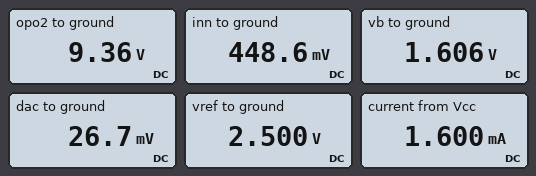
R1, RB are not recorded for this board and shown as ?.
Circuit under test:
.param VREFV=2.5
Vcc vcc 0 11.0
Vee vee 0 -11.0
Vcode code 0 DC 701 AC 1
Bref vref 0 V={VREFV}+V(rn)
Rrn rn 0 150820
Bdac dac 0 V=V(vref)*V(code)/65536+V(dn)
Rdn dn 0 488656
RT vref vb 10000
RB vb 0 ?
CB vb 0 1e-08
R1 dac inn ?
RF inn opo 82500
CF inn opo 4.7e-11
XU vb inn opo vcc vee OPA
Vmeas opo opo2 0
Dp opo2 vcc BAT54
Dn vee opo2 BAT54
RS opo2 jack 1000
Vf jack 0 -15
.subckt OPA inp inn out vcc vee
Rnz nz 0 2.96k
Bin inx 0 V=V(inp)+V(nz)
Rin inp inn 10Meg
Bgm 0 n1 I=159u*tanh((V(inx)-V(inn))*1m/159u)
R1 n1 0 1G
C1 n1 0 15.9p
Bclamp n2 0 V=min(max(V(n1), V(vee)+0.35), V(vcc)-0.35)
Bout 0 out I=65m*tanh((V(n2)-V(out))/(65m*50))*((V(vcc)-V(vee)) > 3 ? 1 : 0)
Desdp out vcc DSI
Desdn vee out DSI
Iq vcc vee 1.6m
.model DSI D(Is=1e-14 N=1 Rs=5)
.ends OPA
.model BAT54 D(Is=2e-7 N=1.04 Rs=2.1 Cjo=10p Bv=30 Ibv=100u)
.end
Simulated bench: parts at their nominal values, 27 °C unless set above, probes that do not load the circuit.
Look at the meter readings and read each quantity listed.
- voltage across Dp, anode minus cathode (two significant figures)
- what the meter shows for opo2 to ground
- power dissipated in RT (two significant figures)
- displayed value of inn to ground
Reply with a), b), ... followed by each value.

a) -1.6 V
b) 9.36 V
c) 80 µW
d) 448.6 mV
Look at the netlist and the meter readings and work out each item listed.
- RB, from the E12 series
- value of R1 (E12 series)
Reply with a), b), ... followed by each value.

a) 18 kΩ
b) 3.9 kΩ
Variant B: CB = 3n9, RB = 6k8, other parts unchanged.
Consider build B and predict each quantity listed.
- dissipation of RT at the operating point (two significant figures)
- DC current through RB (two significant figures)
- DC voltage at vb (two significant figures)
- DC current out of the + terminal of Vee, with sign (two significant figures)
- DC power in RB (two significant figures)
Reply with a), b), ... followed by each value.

a) 220 µW
b) 150 µA
c) 1.0 V
d) -1.6 mA
e) 150 µW
